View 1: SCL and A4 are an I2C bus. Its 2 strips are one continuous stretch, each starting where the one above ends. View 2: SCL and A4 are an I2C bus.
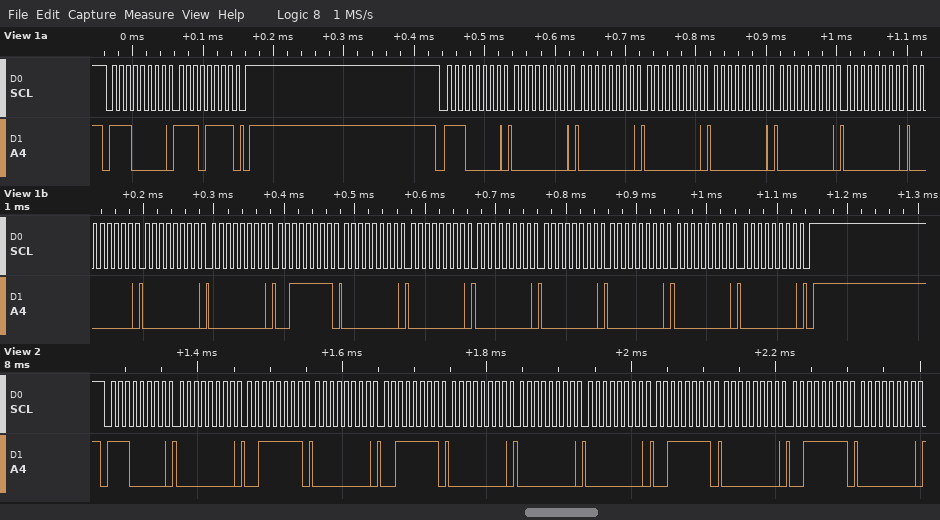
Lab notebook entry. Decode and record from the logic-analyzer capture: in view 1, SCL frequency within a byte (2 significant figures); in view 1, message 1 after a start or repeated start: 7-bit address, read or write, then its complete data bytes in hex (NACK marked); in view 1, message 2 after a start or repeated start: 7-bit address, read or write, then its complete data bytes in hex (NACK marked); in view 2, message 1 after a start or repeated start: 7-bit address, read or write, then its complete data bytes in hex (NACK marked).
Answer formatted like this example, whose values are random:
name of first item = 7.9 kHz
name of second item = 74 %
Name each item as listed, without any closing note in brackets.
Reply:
in view 1, SCL frequency within a byte = 100 kHz
in view 1, message 1 after a start or repeated start: 7-bit address, read or write, then its complete data bytes in hex = 0x70 write: EF
in view 1, message 2 after a start or repeated start: 7-bit address, read or write, then its complete data bytes in hex = 0x70 write: 00 00 00 00 00 00 00 00 00 3F 00 00 00 00 00 00 00
in view 2, message 1 after a start or repeated start: 7-bit address, read or write, then its complete data bytes in hex = 0x70 write: 00 3F 00 3F 00 00 00 3F 00 3F 00
